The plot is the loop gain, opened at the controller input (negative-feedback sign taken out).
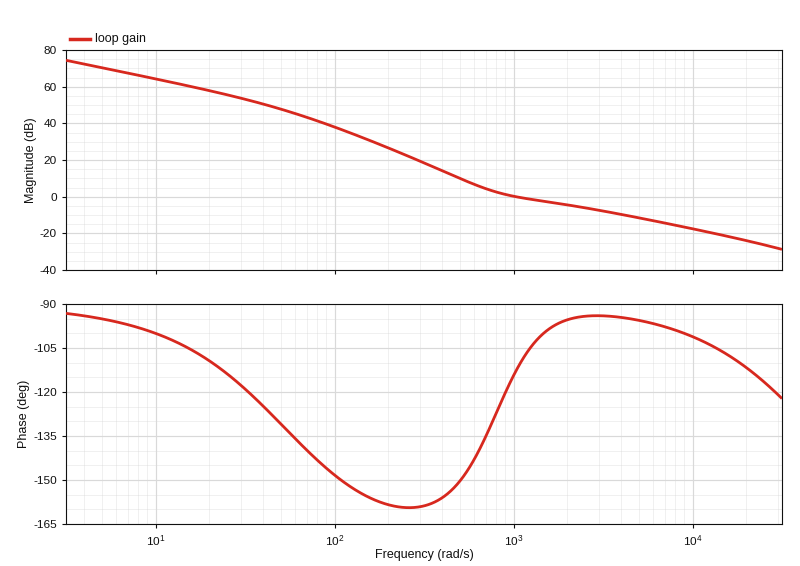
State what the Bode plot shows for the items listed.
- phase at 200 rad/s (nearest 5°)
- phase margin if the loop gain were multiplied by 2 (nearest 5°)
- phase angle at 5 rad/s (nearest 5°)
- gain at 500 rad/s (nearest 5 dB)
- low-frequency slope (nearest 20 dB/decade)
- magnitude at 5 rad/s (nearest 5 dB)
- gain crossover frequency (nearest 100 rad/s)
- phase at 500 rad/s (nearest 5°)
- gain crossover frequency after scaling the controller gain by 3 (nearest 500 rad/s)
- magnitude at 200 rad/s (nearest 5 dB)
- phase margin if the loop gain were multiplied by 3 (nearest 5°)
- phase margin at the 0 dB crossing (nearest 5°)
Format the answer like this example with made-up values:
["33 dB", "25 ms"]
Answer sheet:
["-160°", "85°", "-95°", "10 dB", "-20 dB/decade", "70 dB", "1000 rad/s", "-150°", "4000 rad/s", "25 dB", "85°", "65°"]
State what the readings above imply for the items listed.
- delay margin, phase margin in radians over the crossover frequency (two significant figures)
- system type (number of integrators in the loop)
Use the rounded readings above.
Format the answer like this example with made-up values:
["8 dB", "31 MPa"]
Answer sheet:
["0.0011 s", "1"]
